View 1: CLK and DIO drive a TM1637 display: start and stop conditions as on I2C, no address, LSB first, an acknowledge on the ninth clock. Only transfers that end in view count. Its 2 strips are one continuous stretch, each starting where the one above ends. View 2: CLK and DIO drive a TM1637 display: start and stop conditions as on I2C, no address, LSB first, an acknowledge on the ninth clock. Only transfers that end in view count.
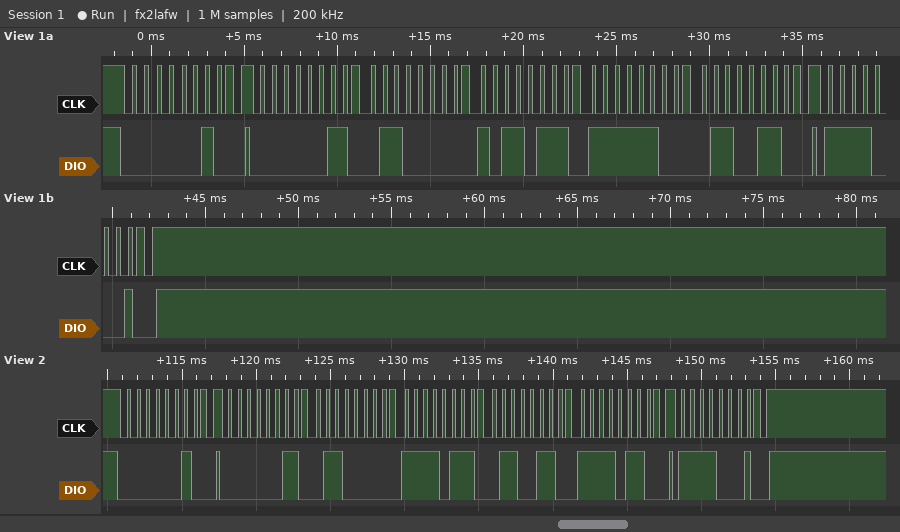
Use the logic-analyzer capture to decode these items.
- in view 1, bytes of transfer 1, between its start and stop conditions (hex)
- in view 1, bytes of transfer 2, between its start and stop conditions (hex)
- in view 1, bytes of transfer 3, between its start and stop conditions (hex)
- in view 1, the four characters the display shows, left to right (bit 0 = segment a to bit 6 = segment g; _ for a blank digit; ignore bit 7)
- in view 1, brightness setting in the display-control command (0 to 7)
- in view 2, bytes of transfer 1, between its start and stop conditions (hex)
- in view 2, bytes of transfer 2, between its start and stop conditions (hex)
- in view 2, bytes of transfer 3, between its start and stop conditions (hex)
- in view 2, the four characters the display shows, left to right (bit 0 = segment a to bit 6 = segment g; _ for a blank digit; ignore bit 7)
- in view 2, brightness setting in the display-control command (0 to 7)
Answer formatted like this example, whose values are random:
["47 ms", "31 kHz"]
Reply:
["40", "C0 06 ED 3F 66", "8F", "1504", "7", "40", "C0 06 EF 66 6F", "8F", "1949", "7"]
